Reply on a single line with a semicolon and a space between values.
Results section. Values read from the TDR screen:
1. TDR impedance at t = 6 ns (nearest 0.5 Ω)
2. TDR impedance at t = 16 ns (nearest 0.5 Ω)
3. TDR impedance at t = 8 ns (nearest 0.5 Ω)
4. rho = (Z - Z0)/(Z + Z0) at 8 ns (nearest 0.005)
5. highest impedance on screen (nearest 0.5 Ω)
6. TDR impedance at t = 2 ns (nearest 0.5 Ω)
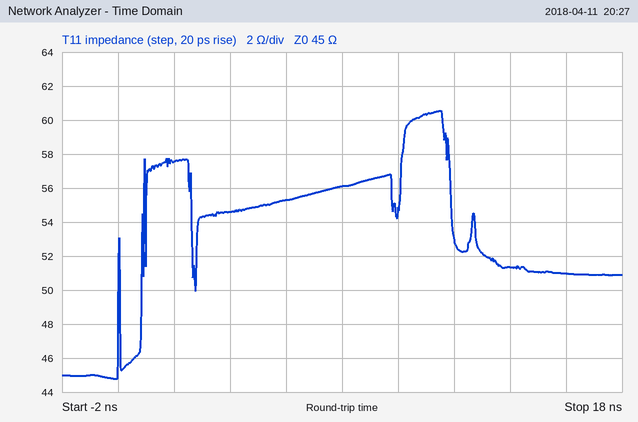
55.5 Ω; 51.0 Ω; 56.0 Ω; +0.110; 60.5 Ω; 57.5 Ω
